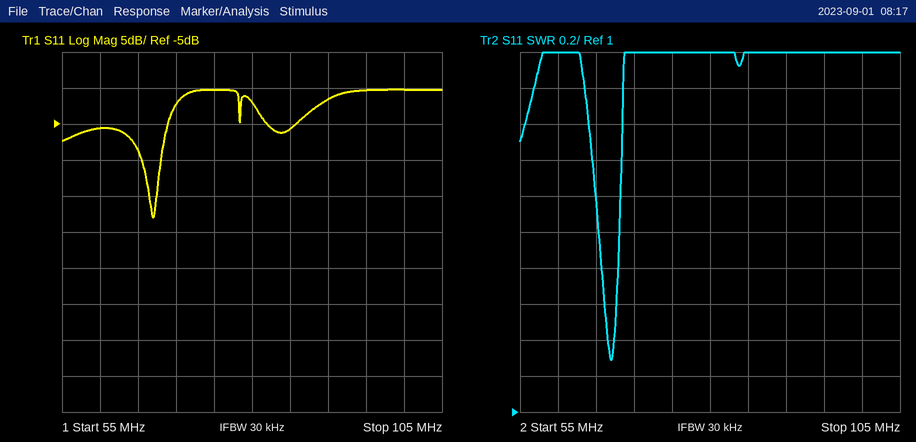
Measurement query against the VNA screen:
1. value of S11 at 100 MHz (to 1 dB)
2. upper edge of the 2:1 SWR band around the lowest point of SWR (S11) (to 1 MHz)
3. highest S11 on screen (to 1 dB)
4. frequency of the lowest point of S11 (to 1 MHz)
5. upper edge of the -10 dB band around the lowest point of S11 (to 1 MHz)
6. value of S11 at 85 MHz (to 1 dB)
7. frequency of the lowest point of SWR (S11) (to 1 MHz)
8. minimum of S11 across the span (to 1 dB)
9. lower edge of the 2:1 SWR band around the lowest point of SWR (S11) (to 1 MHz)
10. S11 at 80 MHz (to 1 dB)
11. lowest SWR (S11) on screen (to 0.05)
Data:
0 dB
68 MHz
0 dB
67 MHz
68 MHz
-6 dB
67 MHz
-18 dB
65 MHz
-2 dB
1.30
